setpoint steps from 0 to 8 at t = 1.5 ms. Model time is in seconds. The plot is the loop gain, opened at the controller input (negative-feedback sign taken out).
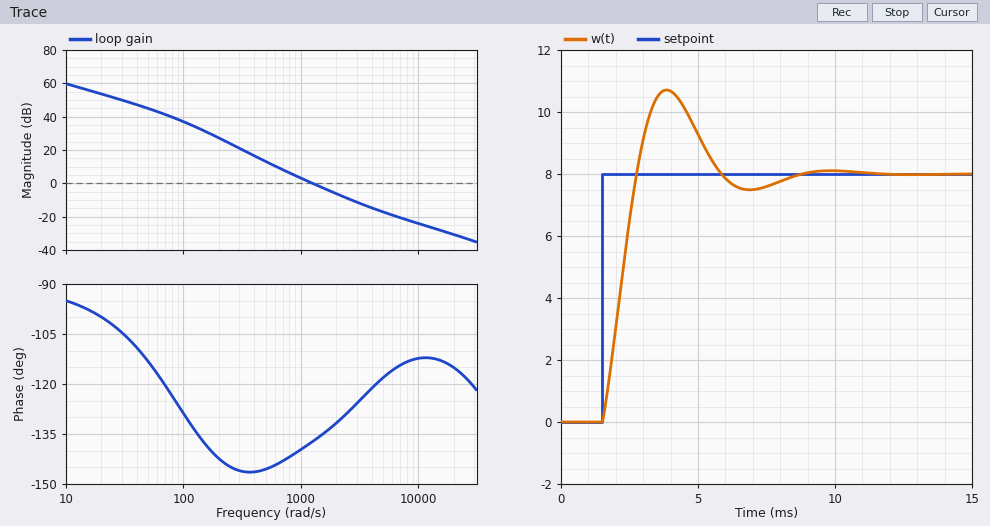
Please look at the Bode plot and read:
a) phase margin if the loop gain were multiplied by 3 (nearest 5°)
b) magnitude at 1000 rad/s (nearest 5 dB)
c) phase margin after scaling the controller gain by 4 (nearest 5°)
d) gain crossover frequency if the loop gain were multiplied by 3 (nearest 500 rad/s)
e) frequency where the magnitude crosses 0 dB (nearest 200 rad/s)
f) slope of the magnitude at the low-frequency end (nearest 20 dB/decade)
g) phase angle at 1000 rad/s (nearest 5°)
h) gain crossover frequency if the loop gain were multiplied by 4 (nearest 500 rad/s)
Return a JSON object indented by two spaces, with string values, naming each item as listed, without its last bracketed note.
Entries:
{
  "phase margin if the loop gain were multiplied by 3": "50°",
  "magnitude at 1000 rad/s": "5 dB",
  "phase margin after scaling the controller gain by 4": "55°",
  "gain crossover frequency if the loop gain were multiplied by 3": "2500 rad/s",
  "frequency where the magnitude crosses 0 dB": "1200 rad/s",
  "slope of the magnitude at the low-frequency end": "-20 dB/decade",
  "phase angle at 1000 rad/s": "-140°",
  "gain crossover frequency if the loop gain were multiplied by 4": "3000 rad/s"
}
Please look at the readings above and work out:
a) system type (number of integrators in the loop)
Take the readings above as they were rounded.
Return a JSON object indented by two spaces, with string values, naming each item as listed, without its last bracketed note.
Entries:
{
  "system type": "1"
}
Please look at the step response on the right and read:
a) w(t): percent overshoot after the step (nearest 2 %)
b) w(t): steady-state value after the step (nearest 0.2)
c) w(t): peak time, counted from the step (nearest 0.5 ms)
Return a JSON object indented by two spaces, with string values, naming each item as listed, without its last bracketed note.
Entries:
{
  "w(t): percent overshoot after the step": "34 %",
  "w(t): steady-state value after the step": "8.0",
  "w(t): peak time, counted from the step": "2.5 ms"
}
